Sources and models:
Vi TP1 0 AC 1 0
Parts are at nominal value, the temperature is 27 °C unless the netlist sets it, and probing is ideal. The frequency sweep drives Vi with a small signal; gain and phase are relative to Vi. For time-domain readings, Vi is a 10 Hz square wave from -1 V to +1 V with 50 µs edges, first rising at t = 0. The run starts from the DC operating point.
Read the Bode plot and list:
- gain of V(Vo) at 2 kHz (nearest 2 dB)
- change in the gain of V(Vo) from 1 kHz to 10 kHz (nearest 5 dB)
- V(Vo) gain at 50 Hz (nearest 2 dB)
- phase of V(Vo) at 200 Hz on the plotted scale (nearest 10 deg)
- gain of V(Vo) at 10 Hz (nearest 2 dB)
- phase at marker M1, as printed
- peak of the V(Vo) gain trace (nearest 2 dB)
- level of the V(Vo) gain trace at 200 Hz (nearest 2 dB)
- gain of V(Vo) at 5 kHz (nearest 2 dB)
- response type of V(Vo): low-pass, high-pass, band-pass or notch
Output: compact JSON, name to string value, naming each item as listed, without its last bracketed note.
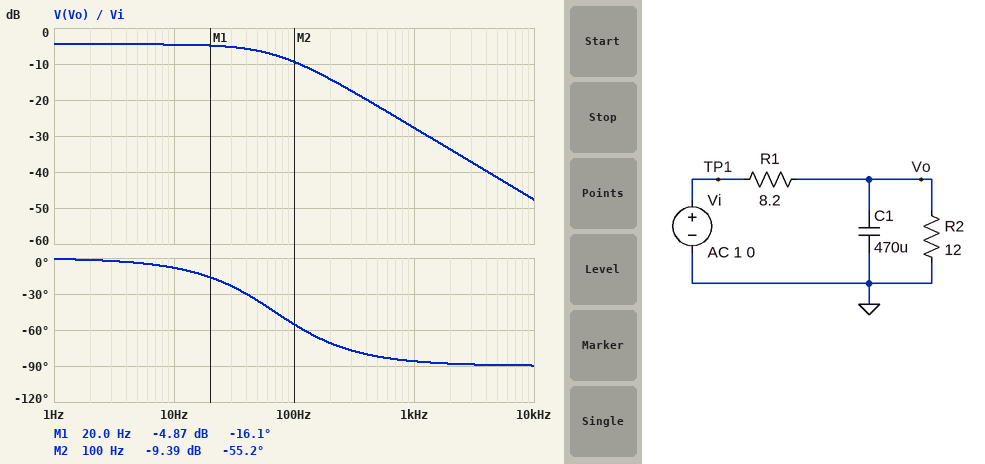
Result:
{"gain of V(Vo) at 2 kHz": "-34 dB", "change in the gain of V(Vo) from 1 kHz to 10 kHz": "-20 dB", "V(Vo) gain at 50 Hz": "-6 dB", "phase of V(Vo) at 200 Hz on the plotted scale": "-70 deg", "gain of V(Vo) at 10 Hz": "-4 dB", "phase at marker M1, as printed": "-16.1 deg", "peak of the V(Vo) gain trace": "-4 dB", "level of the V(Vo) gain trace at 200 Hz": "-14 dB", "gain of V(Vo) at 5 kHz": "-42 dB", "response type of V(Vo): low-pass, high-pass, band-pass or notch": "low-pass"}
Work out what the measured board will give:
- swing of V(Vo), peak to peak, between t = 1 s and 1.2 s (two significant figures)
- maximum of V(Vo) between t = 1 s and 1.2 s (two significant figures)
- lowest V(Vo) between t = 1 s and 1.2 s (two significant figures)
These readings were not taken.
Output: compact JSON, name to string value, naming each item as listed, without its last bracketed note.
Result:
{"swing of V(Vo), peak to peak, between t = 1 s and 1.2 s": "1.2 V", "maximum of V(Vo) between t = 1 s and 1.2 s": "590 mV", "lowest V(Vo) between t = 1 s and 1.2 s": "-590 mV"}
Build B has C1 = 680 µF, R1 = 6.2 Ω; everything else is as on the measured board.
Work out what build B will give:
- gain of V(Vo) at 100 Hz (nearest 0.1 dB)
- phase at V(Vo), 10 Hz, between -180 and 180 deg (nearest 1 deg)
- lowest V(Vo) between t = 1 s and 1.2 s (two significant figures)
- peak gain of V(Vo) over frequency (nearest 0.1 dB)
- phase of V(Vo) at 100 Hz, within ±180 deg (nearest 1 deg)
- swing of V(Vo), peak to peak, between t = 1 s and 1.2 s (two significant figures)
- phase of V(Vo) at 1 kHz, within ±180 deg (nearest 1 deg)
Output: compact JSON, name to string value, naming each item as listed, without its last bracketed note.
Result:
{"gain of V(Vo) at 100 Hz": "-9.7 dB", "phase at V(Vo), 10 Hz, between -180 and 180 deg": "-10 deg", "lowest V(Vo) between t = 1 s and 1.2 s": "-660 mV", "peak gain of V(Vo) over frequency": "-3.6 dB", "phase of V(Vo) at 100 Hz, within ±180 deg": "-60 deg", "swing of V(Vo), peak to peak, between t = 1 s and 1.2 s": "1.3 V", "phase of V(Vo) at 1 kHz, within ±180 deg": "-87 deg"}
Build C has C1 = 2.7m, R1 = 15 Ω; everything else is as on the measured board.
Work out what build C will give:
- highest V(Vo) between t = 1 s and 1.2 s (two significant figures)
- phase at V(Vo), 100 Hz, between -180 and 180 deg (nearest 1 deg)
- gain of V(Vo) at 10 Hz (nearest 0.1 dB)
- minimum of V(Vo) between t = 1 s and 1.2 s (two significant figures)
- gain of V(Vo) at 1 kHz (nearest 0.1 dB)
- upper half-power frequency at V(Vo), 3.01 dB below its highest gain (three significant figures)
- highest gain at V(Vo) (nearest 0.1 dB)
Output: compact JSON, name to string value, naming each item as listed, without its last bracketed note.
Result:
{"highest V(Vo) between t = 1 s and 1.2 s": "390 mV", "phase at V(Vo), 100 Hz, between -180 and 180 deg": "-85 deg", "gain of V(Vo) at 10 Hz": "-10.6 dB", "minimum of V(Vo) between t = 1 s and 1.2 s": "-390 mV", "gain of V(Vo) at 1 kHz": "-48.1 dB", "upper half-power frequency at V(Vo), 3.01 dB below its highest gain": "8.84 Hz", "highest gain at V(Vo)": "-7.0 dB"}
